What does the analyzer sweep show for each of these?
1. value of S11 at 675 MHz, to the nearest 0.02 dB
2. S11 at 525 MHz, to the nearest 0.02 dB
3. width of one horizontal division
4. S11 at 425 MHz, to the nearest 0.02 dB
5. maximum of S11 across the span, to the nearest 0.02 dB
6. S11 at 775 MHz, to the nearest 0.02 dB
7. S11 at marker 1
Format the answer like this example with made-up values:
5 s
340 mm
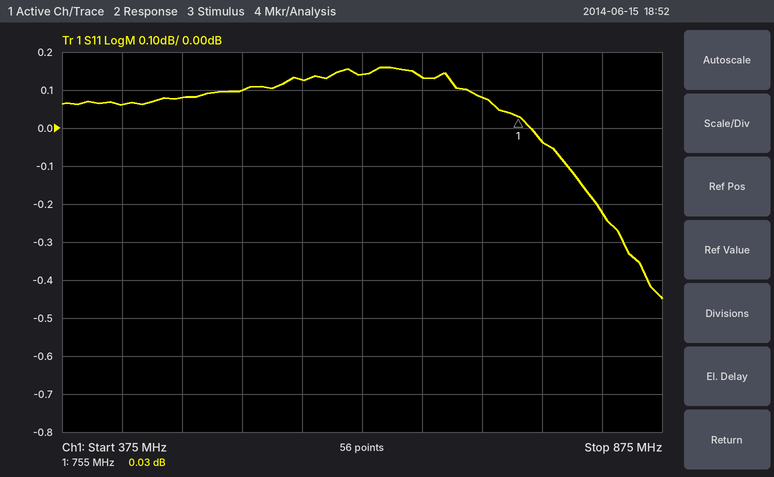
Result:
0.14 dB
0.10 dB
50 MHz
0.06 dB
0.16 dB
-0.04 dB
0.03 dB
